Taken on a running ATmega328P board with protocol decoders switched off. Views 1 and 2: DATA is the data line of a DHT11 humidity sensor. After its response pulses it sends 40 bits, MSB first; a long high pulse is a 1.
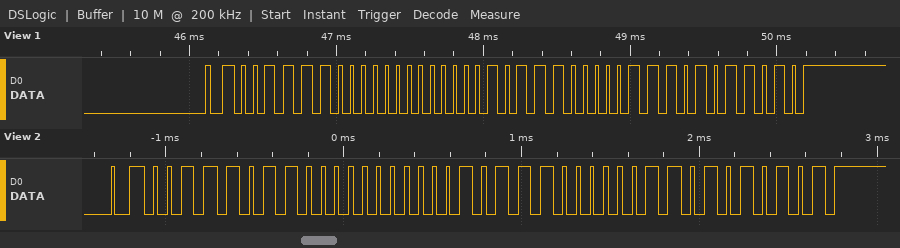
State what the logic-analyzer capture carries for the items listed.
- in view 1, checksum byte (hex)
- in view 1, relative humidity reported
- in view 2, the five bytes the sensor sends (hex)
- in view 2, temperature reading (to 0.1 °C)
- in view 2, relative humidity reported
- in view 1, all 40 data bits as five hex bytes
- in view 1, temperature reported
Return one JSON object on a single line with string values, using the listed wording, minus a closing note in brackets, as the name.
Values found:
{"in view 1, checksum byte": "0x5A", "in view 1, relative humidity reported": "60 %", "in view 2, the five bytes the sensor sends": "3B 00 17 03 55", "in view 2, temperature reading": "23.3 °C", "in view 2, relative humidity reported": "59 %", "in view 1, all 40 data bits as five hex bytes": "3C 00 17 07 5A", "in view 1, temperature reported": "23.7 °C"}
